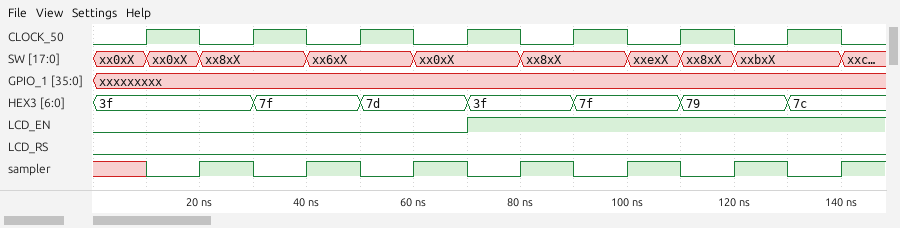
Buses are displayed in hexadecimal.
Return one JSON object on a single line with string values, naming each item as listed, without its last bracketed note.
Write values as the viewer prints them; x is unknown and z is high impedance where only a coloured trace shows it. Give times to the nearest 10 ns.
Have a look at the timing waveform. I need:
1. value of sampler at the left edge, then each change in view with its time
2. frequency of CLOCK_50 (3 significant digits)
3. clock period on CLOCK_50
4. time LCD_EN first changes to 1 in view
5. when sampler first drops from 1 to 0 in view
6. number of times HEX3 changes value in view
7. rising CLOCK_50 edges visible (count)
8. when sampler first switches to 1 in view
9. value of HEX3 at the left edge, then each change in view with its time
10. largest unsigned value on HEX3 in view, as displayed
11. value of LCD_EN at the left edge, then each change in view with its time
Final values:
{"value of sampler at the left edge, then each change in view with its time": "x, 0 at 10 ns, 1 at 20 ns, 0 at 30 ns, 1 at 40 ns, 0 at 50 ns, 1 at 60 ns, 0 at 70 ns, 1 at 80 ns, 0 at 90 ns, 1 at 100 ns, 0 at 110 ns, 1 at 120 ns, 0 at 130 ns, 1 at 140 ns", "frequency of CLOCK_50": "50.0 MHz", "clock period on CLOCK_50": "20 ns", "time LCD_EN first changes to 1 in view": "70 ns", "when sampler first drops from 1 to 0 in view": "30 ns", "number of times HEX3 changes value in view": "6", "rising CLOCK_50 edges visible": "7", "when sampler first switches to 1 in view": "20 ns", "value of HEX3 at the left edge, then each change in view with its time": "3f, 7f at 30 ns, 7d at 50 ns, 3f at 70 ns, 7f at 90 ns, 79 at 110 ns, 7c at 130 ns", "largest unsigned value on HEX3 in view, as displayed": "7f", "value of LCD_EN at the left edge, then each change in view with its time": "0, 1 at 70 ns"}
